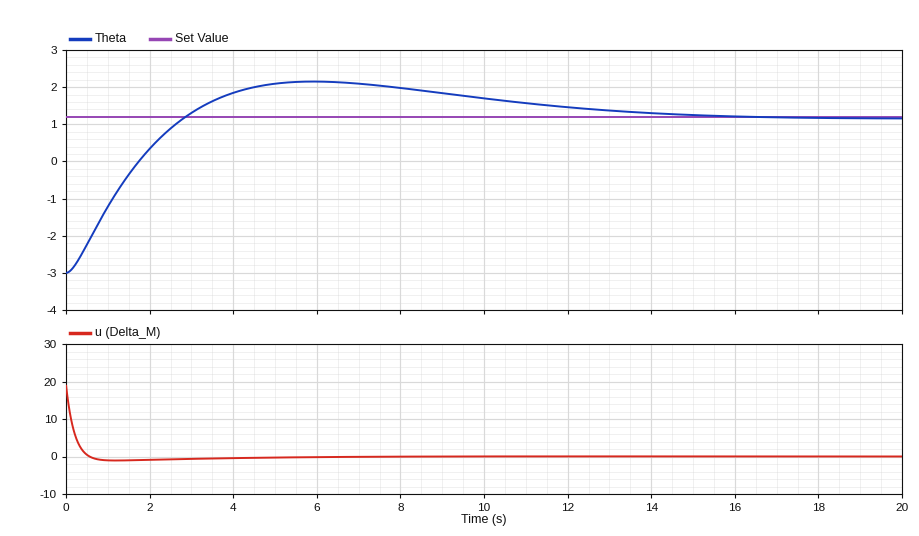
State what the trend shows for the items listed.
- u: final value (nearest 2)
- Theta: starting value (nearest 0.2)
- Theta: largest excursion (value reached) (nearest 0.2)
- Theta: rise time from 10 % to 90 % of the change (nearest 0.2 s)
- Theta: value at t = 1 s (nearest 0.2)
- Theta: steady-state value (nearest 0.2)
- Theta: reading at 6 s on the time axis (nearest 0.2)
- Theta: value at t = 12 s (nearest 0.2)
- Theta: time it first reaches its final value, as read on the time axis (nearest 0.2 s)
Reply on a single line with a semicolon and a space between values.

0; -3.0; 2.2; 2.0 s; -1.2; 1.2; 2.2; 1.4; 2.8 s
